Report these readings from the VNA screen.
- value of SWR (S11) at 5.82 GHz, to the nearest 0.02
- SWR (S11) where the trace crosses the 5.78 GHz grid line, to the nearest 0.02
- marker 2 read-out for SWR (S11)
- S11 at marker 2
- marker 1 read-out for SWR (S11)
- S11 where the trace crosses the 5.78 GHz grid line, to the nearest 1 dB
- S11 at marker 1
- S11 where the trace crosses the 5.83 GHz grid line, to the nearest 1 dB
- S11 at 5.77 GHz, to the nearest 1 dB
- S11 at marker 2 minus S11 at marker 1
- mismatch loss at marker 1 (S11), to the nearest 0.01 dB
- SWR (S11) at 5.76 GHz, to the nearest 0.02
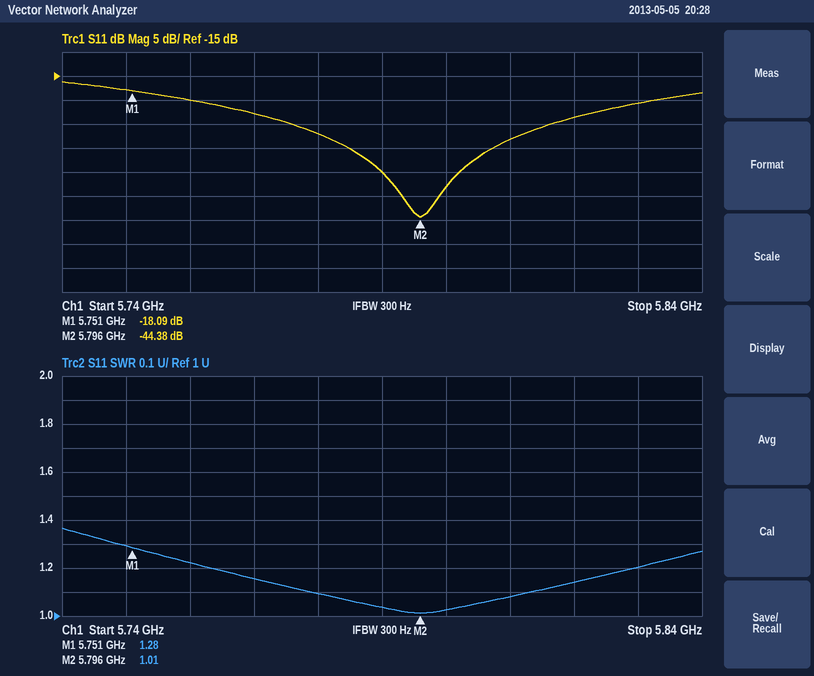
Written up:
1.14
1.10
1.01
-44.38 dB
1.28
-27 dB
-18.09 dB
-21 dB
-23 dB
-26.29 dB
0.07 dB
1.22
